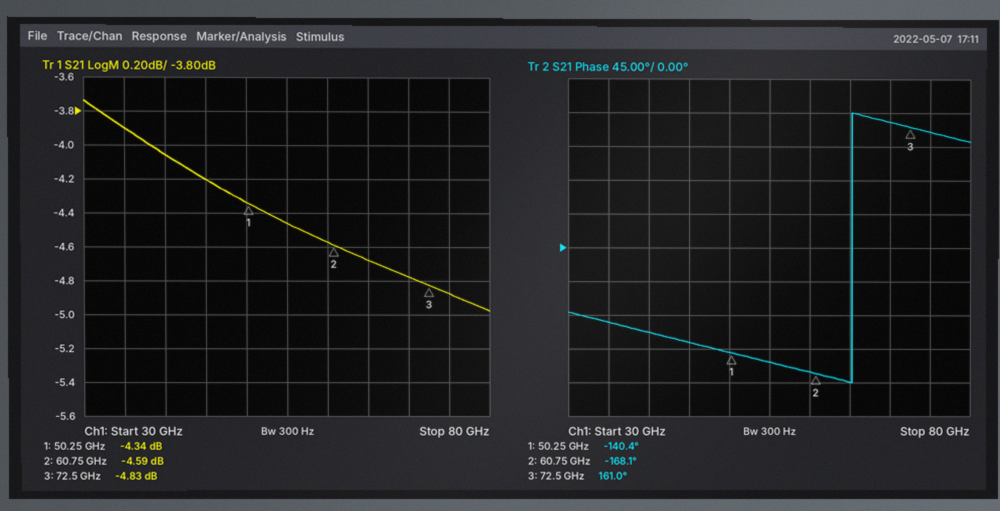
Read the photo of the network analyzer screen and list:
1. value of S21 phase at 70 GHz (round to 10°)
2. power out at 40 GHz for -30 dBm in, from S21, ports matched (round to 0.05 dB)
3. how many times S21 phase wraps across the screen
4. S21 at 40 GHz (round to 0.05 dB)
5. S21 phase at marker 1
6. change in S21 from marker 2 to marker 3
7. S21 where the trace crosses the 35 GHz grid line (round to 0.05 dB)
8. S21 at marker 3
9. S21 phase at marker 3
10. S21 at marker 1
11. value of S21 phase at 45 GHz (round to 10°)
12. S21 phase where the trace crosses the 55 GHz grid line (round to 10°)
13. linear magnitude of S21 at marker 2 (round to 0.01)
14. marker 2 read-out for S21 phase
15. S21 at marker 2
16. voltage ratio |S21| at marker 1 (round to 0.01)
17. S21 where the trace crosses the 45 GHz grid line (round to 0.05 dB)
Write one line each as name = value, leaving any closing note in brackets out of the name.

value of S21 phase at 70 GHz = 170°
power out at 40 GHz for -30 dBm in, from S21, ports matched = -34.05 dBm
how many times S21 phase wraps across the screen = 1
S21 at 40 GHz = -4.05 dB
S21 phase at marker 1 = -140.4°
change in S21 from marker 2 to marker 3 = -0.24 dB
S21 where the trace crosses the 35 GHz grid line = -3.90 dB
S21 at marker 3 = -4.83 dB
S21 phase at marker 3 = 161.0°
S21 at marker 1 = -4.34 dB
value of S21 phase at 45 GHz = -130°
S21 phase where the trace crosses the 55 GHz grid line = -150°
linear magnitude of S21 at marker 2 = 0.59
marker 2 read-out for S21 phase = -168.1°
S21 at marker 2 = -4.59 dB
voltage ratio |S21| at marker 1 = 0.61
S21 where the trace crosses the 45 GHz grid line = -4.20 dB
